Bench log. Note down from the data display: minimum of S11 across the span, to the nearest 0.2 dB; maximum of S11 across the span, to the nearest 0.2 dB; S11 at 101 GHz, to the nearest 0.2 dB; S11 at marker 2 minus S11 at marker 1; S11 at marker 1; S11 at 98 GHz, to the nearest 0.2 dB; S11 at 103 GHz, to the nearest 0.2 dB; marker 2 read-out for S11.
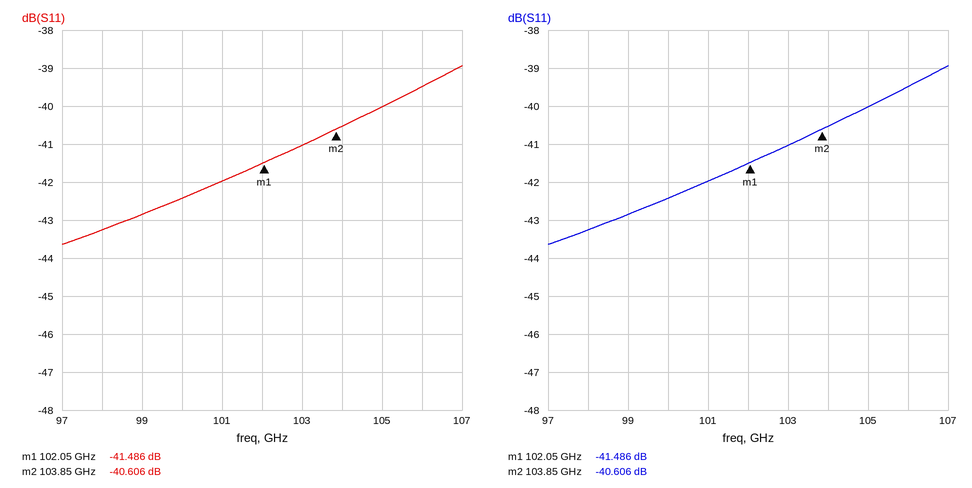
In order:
-43.6 dB
-39.0 dB
-42.0 dB
0.880 dB
-41.486 dB
-43.2 dB
-41.0 dB
-40.606 dB
